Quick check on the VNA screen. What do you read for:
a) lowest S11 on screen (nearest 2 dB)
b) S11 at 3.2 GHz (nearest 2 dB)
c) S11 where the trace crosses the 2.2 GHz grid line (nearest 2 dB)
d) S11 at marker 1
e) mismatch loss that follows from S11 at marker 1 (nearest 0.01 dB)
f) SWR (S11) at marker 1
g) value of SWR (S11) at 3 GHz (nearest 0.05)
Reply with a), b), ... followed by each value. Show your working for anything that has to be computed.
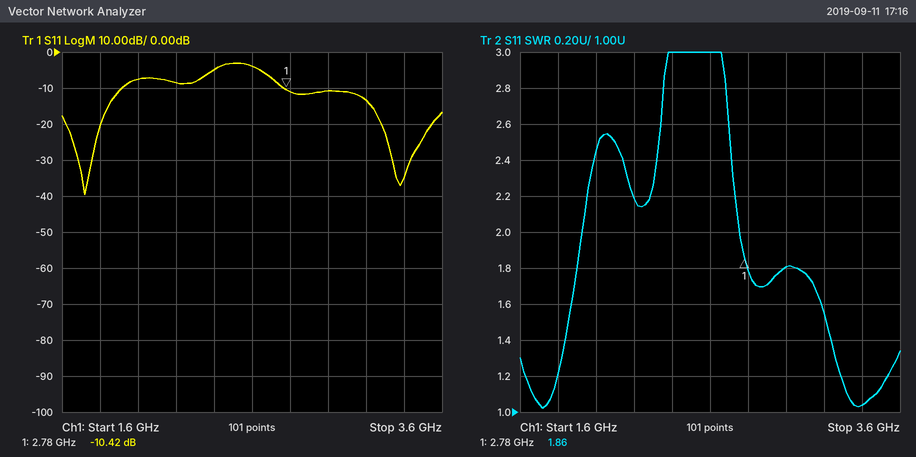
a) -40 dB
b) -14 dB
c) -8 dB
d) -10.42 dB
e) −10 log10(1 − 10^(-10.42/10)) ≈ 0.41 dB
f) 1.86
g) 1.80
